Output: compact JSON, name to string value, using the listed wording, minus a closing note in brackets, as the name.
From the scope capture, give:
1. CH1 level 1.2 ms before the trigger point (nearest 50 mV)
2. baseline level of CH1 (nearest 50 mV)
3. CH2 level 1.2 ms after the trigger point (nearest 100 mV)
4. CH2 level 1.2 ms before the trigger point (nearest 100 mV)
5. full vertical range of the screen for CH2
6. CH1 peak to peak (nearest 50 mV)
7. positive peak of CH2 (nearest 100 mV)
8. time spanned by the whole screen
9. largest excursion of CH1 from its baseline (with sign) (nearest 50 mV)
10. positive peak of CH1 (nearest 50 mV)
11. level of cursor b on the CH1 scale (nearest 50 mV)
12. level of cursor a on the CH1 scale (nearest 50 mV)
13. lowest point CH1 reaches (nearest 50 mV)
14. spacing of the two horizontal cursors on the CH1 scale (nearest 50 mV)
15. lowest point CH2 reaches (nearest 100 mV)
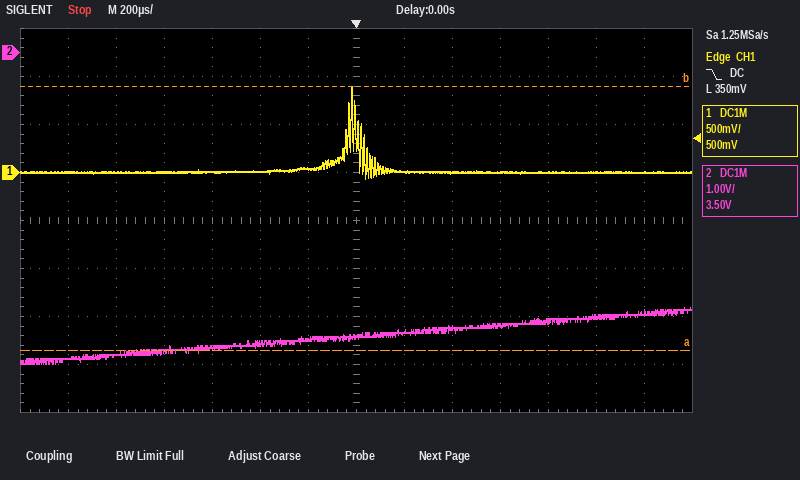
{"CH1 level 1.2 ms before the trigger point": "0 mV", "baseline level of CH1": "0 mV", "CH2 level 1.2 ms after the trigger point": "-5.4 V", "CH2 level 1.2 ms before the trigger point": "-6.4 V", "full vertical range of the screen for CH2": "8 V", "CH1 peak to peak": "950 mV", "positive peak of CH2": "-5.3 V", "time spanned by the whole screen": "2.8 ms", "largest excursion of CH1 from its baseline (with sign)": "+900 mV", "positive peak of CH1": "900 mV", "level of cursor b on the CH1 scale": "900 mV", "level of cursor a on the CH1 scale": "-1.85 V", "lowest point CH1 reaches": "-50 mV", "spacing of the two horizontal cursors on the CH1 scale": "2.75 V", "lowest point CH2 reaches": "-6.5 V"}
